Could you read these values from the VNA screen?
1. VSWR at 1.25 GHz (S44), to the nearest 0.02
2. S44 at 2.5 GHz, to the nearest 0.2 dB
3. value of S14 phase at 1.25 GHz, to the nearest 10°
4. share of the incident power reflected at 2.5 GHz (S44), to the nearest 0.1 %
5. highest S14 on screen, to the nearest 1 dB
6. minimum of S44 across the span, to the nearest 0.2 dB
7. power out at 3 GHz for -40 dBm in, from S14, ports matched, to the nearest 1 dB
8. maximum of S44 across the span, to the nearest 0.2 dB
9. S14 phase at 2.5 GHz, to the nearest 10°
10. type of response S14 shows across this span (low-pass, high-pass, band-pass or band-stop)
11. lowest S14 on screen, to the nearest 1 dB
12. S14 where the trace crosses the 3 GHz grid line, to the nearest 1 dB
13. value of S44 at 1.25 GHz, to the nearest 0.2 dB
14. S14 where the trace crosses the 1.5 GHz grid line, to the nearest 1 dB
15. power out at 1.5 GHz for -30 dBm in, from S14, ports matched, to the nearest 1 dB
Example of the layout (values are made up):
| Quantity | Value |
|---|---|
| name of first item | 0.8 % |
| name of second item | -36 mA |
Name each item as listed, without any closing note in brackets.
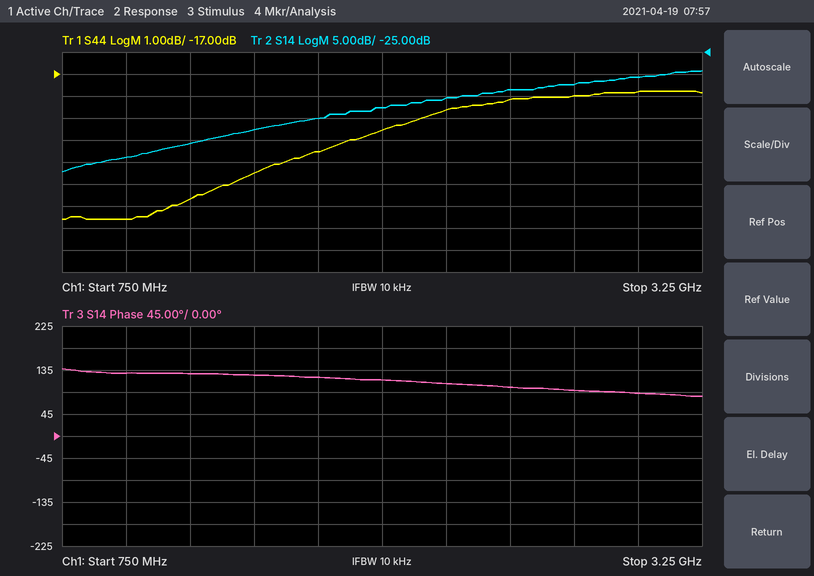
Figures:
| Quantity | Value |
|---|---|
| VSWR at 1.25 GHz (S44), to the nearest 0.02 | 1.16 |
| S44 at 2.5 GHz, to the nearest 0.2 dB | -18.2 dB |
| value of S14 phase at 1.25 GHz, to the nearest 10° | 130° |
| share of the incident power reflected at 2.5 GHz (S44), to the nearest 0.1 % | 1.5 % |
| highest S14 on screen, to the nearest 1 dB | -29 dB |
| minimum of S44 across the span, to the nearest 0.2 dB | -23.6 dB |
| power out at 3 GHz for -40 dBm in, from S14, ports matched, to the nearest 1 dB | -71 dBm |
| maximum of S44 across the span, to the nearest 0.2 dB | -17.8 dB |
| S14 phase at 2.5 GHz, to the nearest 10° | 100° |
| type of response S14 shows across this span | high-pass |
| lowest S14 on screen, to the nearest 1 dB | -52 dB |
| S14 where the trace crosses the 3 GHz grid line, to the nearest 1 dB | -31 dB |
| value of S44 at 1.25 GHz, to the nearest 0.2 dB | -22.6 dB |
| S14 where the trace crosses the 1.5 GHz grid line, to the nearest 1 dB | -43 dB |
| power out at 1.5 GHz for -30 dBm in, from S14, ports matched, to the nearest 1 dB | -73 dBm |
